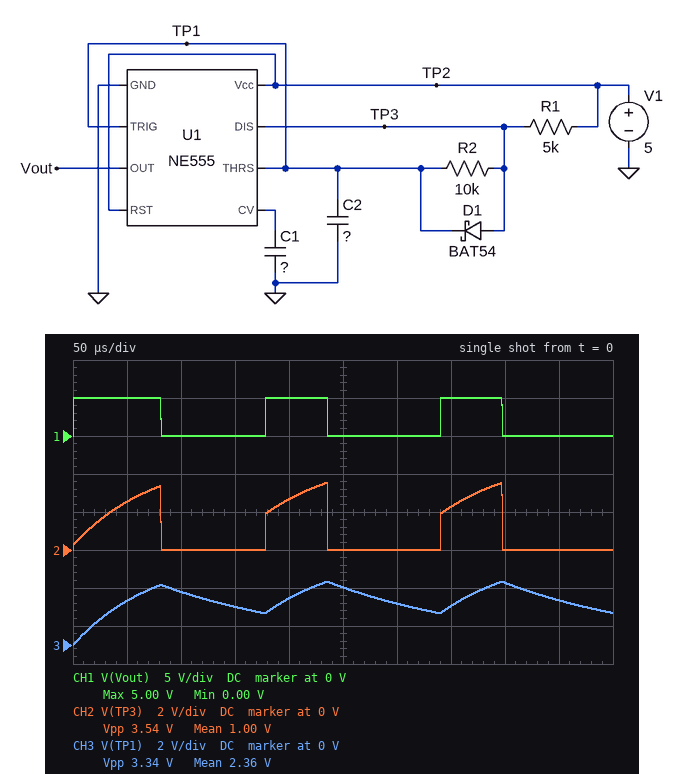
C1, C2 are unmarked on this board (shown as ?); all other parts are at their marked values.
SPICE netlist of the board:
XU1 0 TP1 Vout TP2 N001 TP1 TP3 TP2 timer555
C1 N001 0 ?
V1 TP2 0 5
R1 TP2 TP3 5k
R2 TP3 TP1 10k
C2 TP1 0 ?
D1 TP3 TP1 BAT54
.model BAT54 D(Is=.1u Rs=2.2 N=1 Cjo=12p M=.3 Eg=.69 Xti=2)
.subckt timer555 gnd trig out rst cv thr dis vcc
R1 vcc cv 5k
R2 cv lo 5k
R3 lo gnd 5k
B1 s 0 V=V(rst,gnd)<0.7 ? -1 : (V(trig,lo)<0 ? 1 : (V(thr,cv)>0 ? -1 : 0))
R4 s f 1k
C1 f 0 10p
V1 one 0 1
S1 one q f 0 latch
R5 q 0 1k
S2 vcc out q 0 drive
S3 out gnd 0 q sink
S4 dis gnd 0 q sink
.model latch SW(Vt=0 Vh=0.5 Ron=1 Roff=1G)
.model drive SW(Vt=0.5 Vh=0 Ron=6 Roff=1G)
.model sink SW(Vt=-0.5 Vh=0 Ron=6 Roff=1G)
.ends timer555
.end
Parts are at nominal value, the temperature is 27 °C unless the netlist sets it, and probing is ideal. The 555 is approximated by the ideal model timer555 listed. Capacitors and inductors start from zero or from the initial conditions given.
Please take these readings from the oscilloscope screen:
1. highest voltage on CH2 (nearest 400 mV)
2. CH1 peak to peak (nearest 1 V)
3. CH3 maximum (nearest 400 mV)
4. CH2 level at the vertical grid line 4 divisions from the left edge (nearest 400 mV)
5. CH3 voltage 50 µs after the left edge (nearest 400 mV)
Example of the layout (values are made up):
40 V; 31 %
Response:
3.6 V; 5 V; 3.2 V; 2.8 V; 2.4 V
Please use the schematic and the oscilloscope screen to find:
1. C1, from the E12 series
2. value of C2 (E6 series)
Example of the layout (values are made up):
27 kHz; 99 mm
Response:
8.2 nF; 15 nF
